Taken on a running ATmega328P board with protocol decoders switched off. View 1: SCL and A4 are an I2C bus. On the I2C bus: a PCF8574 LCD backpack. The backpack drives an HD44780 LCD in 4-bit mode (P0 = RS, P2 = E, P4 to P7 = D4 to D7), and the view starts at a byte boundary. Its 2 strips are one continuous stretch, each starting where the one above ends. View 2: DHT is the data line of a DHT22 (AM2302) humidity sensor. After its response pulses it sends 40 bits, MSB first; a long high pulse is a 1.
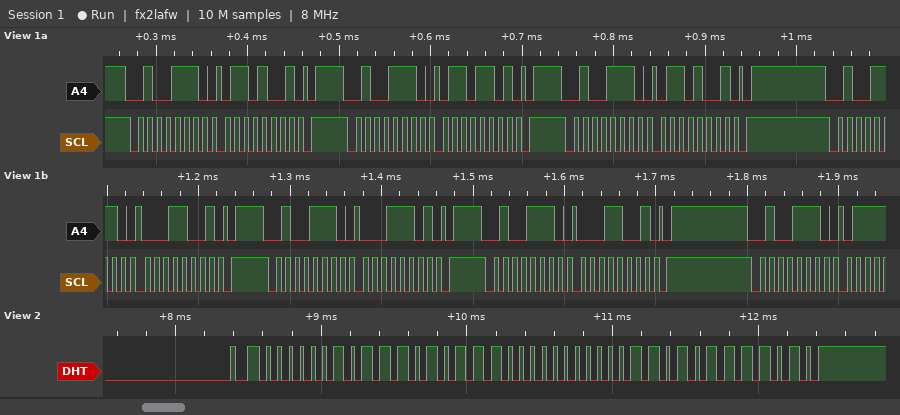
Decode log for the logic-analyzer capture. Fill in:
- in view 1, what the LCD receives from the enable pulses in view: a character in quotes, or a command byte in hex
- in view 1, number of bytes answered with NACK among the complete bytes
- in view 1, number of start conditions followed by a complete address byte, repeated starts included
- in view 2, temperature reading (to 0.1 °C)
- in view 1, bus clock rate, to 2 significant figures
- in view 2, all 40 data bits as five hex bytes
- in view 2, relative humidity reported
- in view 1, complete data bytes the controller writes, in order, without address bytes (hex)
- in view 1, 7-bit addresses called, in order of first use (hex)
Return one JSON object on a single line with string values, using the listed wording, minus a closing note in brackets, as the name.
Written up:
{"in view 1, what the LCD receives from the enable pulses in view: a character in quotes, or a command byte in hex": "'a'", "in view 1, number of bytes answered with NACK among the complete bytes": "0", "in view 1, number of start conditions followed by a complete address byte, repeated starts included": "7", "in view 2, temperature reading": "-1.3 °C", "in view 1, bus clock rate, to 2 significant figures": "100 kHz", "in view 2, all 40 data bits as five hex bytes": "02 EB 80 0D 7A", "in view 2, relative humidity reported": "74.7 %", "in view 1, complete data bytes the controller writes, in order, without address bytes": "69 6D 69 19 1D 19", "in view 1, 7-bit addresses called, in order of first use": "0x27"}
